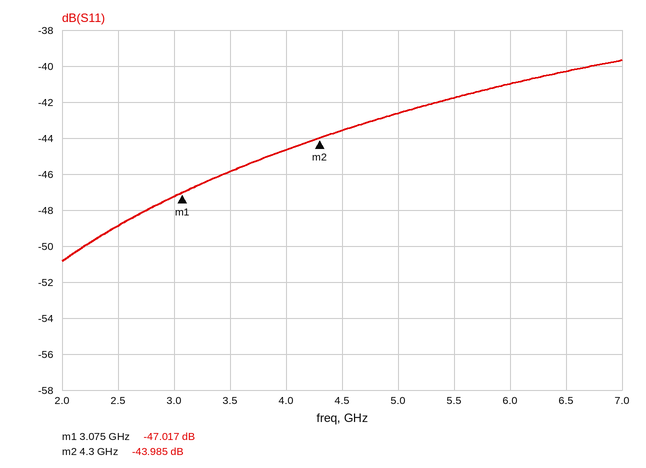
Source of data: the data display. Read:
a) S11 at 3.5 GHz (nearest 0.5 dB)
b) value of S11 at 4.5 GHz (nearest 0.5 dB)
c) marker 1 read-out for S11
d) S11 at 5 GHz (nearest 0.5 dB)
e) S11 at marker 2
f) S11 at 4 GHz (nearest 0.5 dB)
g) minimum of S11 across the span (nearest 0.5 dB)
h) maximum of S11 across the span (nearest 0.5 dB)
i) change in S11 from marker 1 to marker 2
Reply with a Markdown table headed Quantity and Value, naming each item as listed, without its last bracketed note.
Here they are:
| Quantity | Value |
|---|---|
| S11 at 3.5 GHz | -46.0 dB |
| value of S11 at 4.5 GHz | -43.5 dB |
| marker 1 read-out for S11 | -47.017 dB |
| S11 at 5 GHz | -42.5 dB |
| S11 at marker 2 | -43.985 dB |
| S11 at 4 GHz | -44.5 dB |
| minimum of S11 across the span | -51.0 dB |
| maximum of S11 across the span | -39.5 dB |
| change in S11 from marker 1 to marker 2 | 3.032 dB |
